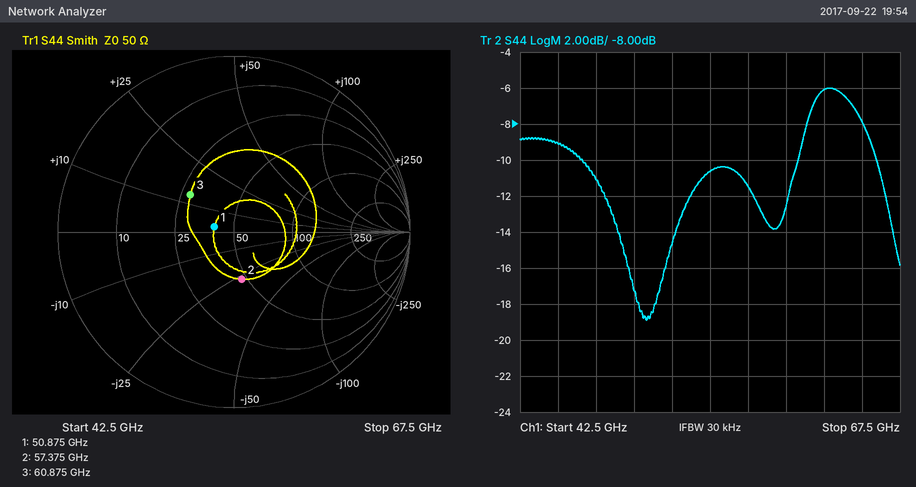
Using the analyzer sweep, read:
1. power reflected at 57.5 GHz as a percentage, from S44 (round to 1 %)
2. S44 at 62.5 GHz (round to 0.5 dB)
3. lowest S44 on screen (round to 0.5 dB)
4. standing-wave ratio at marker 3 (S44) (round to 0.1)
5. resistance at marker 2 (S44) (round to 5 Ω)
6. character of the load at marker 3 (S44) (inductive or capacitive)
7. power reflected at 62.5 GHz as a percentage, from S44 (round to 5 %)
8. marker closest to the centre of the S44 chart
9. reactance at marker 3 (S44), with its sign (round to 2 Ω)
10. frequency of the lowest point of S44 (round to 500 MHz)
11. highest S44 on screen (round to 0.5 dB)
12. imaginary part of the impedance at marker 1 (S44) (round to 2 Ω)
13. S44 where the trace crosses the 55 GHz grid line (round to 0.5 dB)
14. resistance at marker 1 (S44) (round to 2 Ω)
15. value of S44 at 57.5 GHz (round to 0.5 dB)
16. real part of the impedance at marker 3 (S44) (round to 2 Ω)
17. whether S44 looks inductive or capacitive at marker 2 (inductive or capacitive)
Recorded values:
7 %
-6.0 dB
-19.0 dB
2.0
45 Ω
inductive
25 %
marker 1
+14 Ω
51.0 GHz
-6.0 dB
+2 Ω
-10.5 dB
40 Ω
-11.5 dB
28 Ω
capacitive
